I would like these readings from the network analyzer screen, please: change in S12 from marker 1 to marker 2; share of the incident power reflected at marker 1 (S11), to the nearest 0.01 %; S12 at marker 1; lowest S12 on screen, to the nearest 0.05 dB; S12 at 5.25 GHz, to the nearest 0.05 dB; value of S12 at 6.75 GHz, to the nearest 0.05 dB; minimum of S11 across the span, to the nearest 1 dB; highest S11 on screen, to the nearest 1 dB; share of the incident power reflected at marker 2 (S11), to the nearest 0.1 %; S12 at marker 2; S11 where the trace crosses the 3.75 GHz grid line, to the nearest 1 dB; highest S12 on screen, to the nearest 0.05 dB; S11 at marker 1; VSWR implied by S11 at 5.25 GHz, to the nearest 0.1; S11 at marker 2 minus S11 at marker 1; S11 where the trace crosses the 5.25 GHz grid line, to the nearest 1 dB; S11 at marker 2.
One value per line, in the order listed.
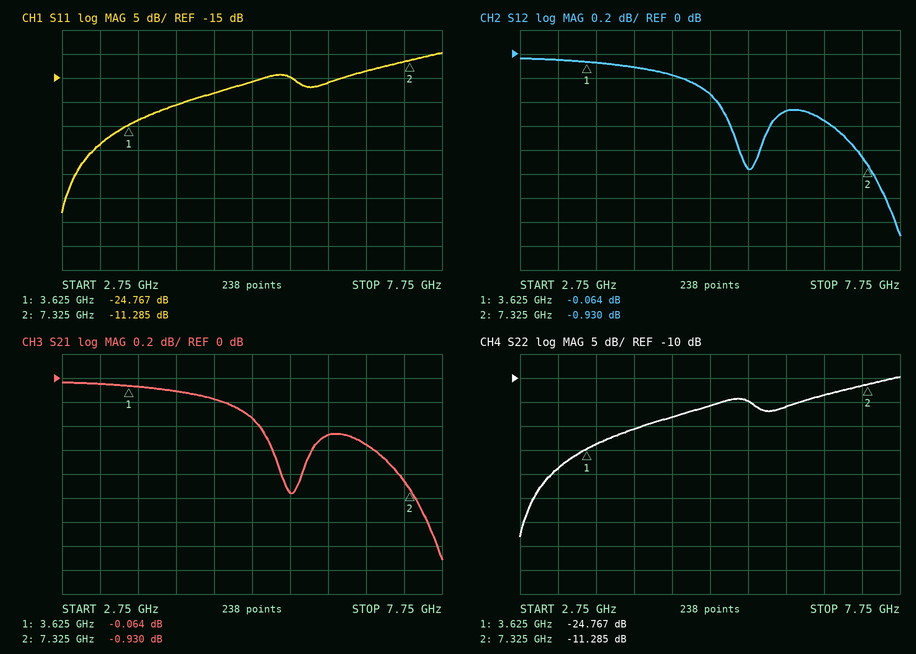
-0.866 dB
0.33 %
-0.064 dB
-1.50 dB
-0.35 dB
-0.55 dB
-43 dB
-10 dB
7.4 %
-0.930 dB
-24 dB
-0.05 dB
-24.767 dB
1.4
13.482 dB
-16 dB
-11.285 dB
